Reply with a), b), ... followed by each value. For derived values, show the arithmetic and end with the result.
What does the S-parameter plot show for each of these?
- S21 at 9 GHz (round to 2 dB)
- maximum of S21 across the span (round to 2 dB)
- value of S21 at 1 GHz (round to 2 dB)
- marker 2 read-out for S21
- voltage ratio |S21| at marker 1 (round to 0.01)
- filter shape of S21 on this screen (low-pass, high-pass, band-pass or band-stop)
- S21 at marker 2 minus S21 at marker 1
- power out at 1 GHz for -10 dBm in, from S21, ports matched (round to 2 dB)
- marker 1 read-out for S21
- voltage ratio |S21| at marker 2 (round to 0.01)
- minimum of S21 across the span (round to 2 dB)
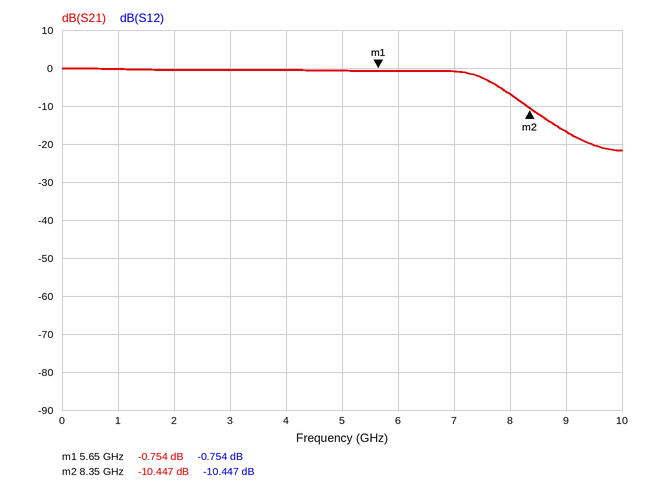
a) -16 dB
b) 0 dB
c) 0 dB
d) -10.447 dB
e) 10^(-0.754/20) ≈ 0.92
f) low-pass
g) -10.447 − (-0.754) = -9.693 dB
h) -10 dBm + (0 dB) = -10 dBm
i) -0.754 dB
j) 10^(-10.447/20) ≈ 0.30
k) -22 dB
